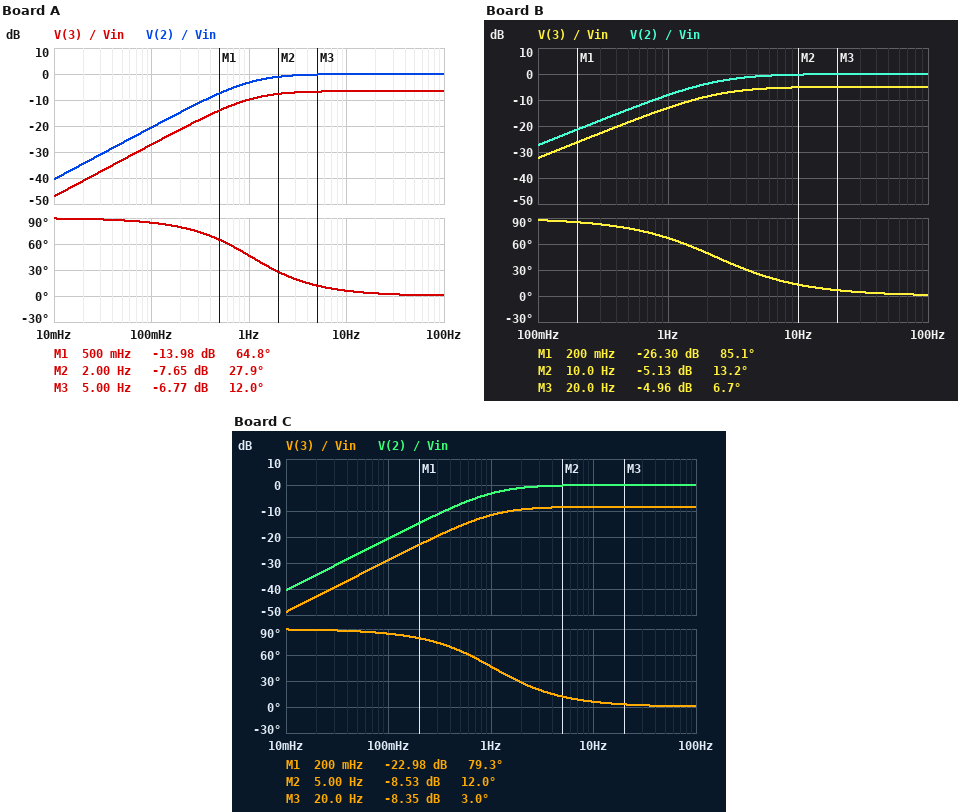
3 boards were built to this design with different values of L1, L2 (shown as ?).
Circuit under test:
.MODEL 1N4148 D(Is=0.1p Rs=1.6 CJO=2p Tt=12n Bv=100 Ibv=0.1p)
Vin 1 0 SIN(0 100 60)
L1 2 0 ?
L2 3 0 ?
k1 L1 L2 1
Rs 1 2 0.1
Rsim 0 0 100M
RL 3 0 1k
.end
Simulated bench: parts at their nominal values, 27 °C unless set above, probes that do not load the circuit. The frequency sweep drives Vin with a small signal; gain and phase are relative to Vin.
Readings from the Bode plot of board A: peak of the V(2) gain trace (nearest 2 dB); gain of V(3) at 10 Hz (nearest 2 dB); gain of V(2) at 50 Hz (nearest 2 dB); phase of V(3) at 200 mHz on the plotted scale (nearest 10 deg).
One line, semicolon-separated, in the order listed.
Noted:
0 dB; -6 dB; 0 dB; 80 deg
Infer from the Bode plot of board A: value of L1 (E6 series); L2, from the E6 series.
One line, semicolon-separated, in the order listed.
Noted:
15 mH; 3.3 mH
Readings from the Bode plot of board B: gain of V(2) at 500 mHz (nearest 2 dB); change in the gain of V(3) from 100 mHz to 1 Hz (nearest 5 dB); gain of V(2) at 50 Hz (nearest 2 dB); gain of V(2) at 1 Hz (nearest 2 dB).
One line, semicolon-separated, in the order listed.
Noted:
-14 dB; 20 dB; 0 dB; -8 dB
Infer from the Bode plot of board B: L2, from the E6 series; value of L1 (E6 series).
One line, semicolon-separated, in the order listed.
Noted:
2.2 mH; 6.8 mH
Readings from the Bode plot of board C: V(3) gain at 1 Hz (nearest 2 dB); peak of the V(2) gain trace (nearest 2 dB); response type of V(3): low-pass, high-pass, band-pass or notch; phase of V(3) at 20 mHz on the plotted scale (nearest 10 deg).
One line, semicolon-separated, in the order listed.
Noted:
-12 dB; 0 dB; high-pass; 90 deg
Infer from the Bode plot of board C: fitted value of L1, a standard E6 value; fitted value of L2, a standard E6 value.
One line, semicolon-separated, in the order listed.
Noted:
15 mH; 2.2 mH
